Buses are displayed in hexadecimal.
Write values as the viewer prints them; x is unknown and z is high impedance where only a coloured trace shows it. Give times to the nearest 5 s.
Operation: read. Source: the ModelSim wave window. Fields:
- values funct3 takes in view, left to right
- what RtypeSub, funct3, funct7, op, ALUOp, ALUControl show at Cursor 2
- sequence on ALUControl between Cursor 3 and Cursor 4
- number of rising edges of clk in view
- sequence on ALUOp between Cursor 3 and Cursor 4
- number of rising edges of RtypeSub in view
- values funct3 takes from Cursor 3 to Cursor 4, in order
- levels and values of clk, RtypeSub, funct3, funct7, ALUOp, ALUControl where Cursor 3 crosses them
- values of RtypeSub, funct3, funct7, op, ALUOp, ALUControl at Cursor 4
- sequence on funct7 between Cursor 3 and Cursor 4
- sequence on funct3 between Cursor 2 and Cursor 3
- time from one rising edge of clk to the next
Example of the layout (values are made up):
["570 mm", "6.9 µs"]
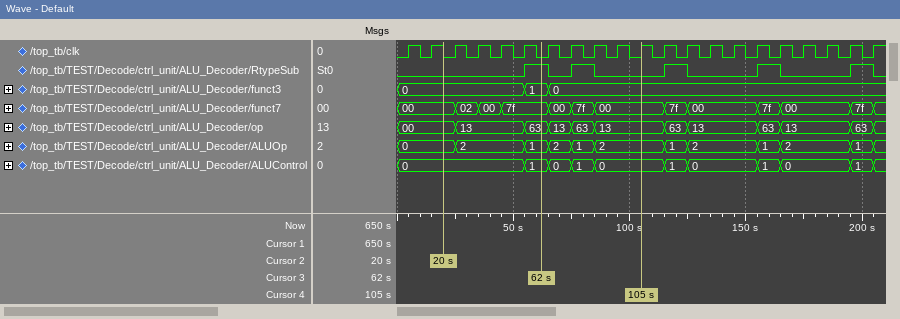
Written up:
["0, 1, 0", "RtypeSub=0, funct3=0, funct7=00, op=00, ALUOp=0, ALUControl=0", "1, 0, 1, 0", "21", "1, 2, 1, 2", "5", "1, 0", "clk=0, RtypeSub=1, funct3=1, funct7=7f, ALUOp=1, ALUControl=1", "RtypeSub=0, funct3=0, funct7=00, op=13, ALUOp=2, ALUControl=0", "7f, 00, 7f, 00", "0, 1", "10 s"]
